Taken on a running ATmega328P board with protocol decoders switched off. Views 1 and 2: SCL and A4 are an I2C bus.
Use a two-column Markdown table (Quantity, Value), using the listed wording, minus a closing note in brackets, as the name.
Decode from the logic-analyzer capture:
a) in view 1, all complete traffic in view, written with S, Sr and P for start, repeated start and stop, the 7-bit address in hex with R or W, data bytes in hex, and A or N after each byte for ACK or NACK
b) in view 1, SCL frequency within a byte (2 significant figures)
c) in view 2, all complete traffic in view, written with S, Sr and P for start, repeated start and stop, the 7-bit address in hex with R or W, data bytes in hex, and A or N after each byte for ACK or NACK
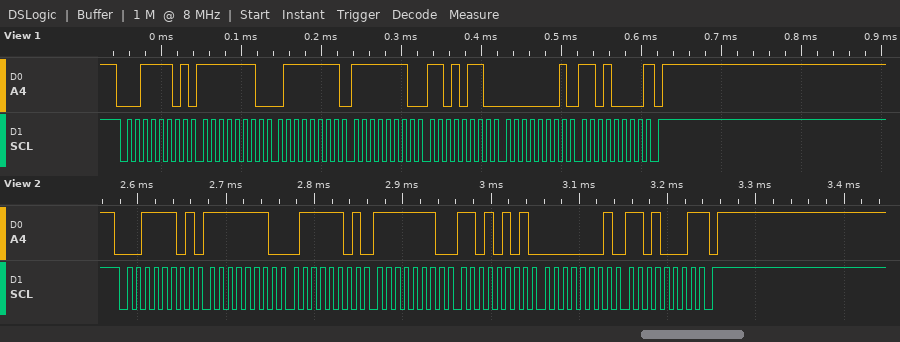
| Quantity | Value |
|---|---|
| in view 1, all complete traffic in view, written with S, Sr and P for start, repeated start and stop, the 7-bit address in hex with R or W, data bytes in hex, and A or N after each byte for ACK or NACK | S 1ER A FE A 7F A FE A D6 A 01 A D0 N P |
| in view 1, SCL frequency within a byte | 100 kHz |
| in view 2, all complete traffic in view, written with S, Sr and P for start, repeated start and stop, the 7-bit address in hex with R or W, data bytes in hex, and A or N after each byte for ACK or NACK | S 1ER A FE A 7D A FE A D5 A 01 A D1 N P |
